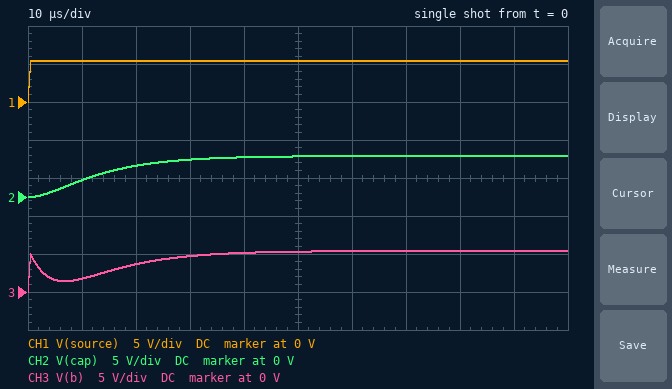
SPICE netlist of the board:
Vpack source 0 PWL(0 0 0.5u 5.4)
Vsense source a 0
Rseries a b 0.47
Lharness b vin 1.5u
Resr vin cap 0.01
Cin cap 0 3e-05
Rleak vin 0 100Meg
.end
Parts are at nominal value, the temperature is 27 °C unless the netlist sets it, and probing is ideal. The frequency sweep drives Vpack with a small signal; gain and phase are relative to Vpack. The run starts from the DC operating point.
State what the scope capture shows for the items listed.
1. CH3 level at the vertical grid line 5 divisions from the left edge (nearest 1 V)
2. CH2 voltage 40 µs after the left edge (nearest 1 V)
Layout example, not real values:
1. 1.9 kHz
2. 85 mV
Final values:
1. 5 V
2. 5 V
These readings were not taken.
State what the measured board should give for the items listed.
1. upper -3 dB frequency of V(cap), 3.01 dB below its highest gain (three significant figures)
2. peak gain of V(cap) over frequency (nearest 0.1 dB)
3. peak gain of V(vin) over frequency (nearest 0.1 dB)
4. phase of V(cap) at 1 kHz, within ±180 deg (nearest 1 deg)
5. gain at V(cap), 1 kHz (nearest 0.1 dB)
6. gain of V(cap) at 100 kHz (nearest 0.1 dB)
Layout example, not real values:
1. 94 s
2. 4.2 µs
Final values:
1. 13.8 kHz
2. 0 dB
3. 0 dB
4. -5 deg
5. 0 dB
6. -25.6 dB
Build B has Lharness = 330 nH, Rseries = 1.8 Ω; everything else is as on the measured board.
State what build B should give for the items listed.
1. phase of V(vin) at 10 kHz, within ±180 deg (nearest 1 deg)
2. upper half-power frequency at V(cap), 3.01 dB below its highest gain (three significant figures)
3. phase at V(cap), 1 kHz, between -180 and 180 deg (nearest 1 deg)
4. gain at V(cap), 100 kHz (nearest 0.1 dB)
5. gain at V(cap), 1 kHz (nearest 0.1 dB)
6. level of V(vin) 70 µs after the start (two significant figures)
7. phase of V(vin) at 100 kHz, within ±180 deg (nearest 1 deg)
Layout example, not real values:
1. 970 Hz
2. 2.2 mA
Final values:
1. -73 deg
2. 2.94 kHz
3. -19 deg
4. -30.7 dB
5. -0.5 dB
6. 3.9 V
7. -84 deg
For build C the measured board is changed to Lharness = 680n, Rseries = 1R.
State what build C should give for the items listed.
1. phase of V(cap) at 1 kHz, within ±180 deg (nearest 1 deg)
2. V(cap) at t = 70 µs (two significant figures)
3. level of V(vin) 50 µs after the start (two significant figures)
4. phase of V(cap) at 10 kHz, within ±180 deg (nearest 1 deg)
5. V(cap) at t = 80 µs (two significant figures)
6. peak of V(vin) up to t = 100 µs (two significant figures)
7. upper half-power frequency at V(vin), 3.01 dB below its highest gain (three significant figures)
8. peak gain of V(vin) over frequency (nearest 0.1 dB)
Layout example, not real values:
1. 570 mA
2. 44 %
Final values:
1. -11 deg
2. 4.9 V
3. 4.4 V
4. -64 deg
5. 5.0 V
6. 5.2 V
7. 5.37 kHz
8. 0 dB
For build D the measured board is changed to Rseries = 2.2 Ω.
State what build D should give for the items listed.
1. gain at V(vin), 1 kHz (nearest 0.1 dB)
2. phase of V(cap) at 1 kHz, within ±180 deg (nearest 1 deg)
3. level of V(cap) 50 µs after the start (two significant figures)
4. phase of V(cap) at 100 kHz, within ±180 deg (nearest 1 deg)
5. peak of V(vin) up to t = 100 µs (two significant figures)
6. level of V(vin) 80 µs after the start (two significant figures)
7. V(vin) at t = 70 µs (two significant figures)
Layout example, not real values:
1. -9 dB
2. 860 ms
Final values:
1. -0.7 dB
2. -23 deg
3. 2.8 V
4. -112 deg
5. 4.2 V
6. 3.8 V
7. 3.5 V
